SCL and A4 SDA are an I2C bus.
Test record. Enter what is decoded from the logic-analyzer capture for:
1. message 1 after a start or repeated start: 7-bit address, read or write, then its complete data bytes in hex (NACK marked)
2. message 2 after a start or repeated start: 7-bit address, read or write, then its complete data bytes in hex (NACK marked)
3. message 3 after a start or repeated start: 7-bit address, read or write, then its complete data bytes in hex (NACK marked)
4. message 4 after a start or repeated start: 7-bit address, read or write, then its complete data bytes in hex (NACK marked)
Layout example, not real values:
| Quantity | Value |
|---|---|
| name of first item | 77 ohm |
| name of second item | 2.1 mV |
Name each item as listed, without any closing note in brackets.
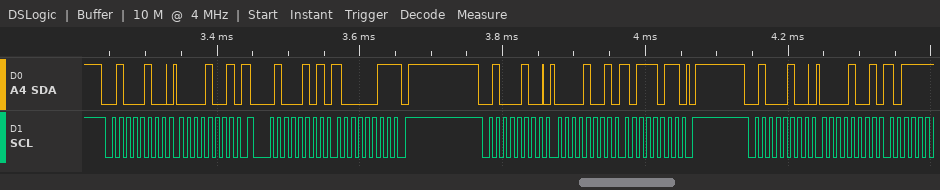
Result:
| Quantity | Value |
|---|---|
| message 1 after a start or repeated start: 7-bit address, read or write, then its complete data bytes in hex | 0x22 write: 09 |
| message 2 after a start or repeated start: 7-bit address, read or write, then its complete data bytes in hex | 0x22 read: 83 NACK |
| message 3 after a start or repeated start: 7-bit address, read or write, then its complete data bytes in hex | 0x22 write: 09 BB |
| message 4 after a start or repeated start: 7-bit address, read or write, then its complete data bytes in hex | 0x22 write: 09 |
